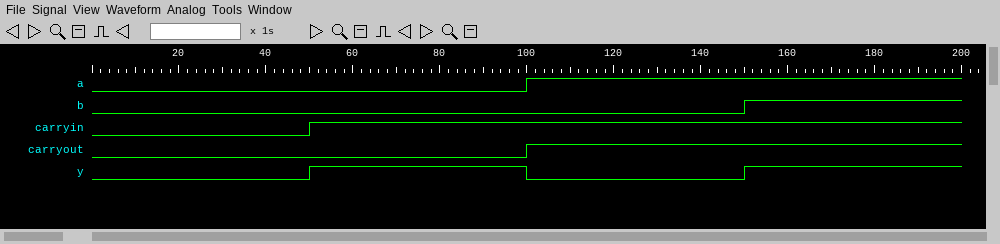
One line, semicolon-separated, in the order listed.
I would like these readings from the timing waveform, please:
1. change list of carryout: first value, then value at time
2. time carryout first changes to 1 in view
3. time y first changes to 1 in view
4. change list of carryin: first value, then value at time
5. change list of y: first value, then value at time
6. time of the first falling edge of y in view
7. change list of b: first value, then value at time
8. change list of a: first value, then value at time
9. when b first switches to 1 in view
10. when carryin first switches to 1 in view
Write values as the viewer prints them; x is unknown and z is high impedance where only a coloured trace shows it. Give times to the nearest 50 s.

0, 1 at 100 s; 100 s; 50 s; 0, 1 at 50 s; 0, 1 at 50 s, 0 at 100 s, 1 at 150 s; 100 s; 0, 1 at 150 s; 0, 1 at 100 s; 150 s; 50 s
